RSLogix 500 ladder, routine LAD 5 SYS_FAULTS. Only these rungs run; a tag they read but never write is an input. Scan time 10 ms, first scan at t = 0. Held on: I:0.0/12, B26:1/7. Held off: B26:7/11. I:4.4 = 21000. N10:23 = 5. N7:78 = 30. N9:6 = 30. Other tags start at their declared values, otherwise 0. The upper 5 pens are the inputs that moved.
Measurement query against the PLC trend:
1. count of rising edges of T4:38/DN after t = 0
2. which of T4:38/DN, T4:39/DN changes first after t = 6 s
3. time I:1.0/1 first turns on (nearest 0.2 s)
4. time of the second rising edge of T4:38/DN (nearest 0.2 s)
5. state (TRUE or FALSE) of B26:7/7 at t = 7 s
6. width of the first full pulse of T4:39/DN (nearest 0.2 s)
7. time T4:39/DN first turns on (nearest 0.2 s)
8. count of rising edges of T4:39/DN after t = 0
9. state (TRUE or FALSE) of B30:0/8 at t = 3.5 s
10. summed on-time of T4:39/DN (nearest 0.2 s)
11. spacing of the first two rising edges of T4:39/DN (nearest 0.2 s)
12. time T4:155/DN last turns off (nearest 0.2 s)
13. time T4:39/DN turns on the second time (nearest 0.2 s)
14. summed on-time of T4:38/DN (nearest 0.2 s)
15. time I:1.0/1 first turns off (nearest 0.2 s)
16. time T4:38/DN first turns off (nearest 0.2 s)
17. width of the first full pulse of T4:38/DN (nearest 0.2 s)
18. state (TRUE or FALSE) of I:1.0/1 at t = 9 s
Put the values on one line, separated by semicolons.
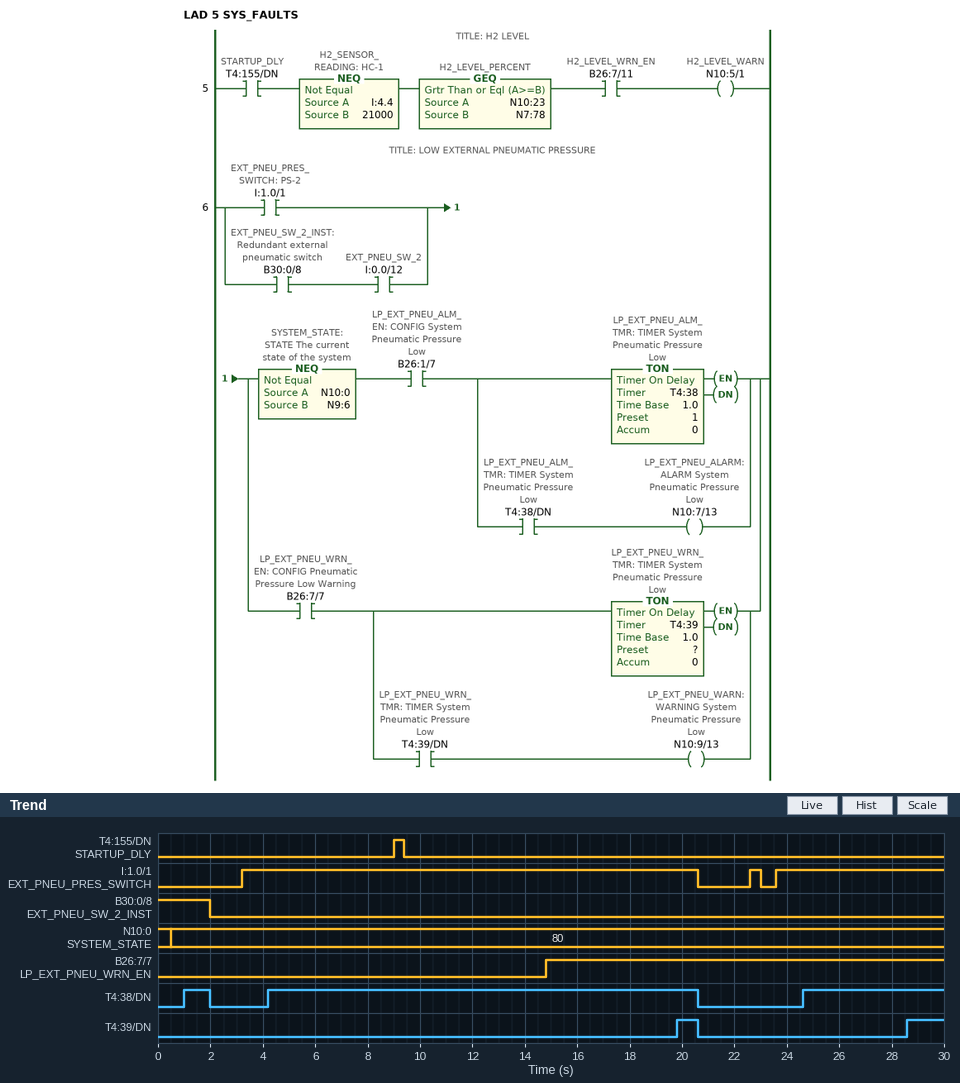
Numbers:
3; T4:39/DN; 3.2 s; 4.2 s; FALSE; 0.8 s; 19.8 s; 2; FALSE; 2.2 s; 8.8 s; 9.4 s; 28.6 s; 22.8 s; 20.6 s; 2.0 s; 1.0 s; TRUE
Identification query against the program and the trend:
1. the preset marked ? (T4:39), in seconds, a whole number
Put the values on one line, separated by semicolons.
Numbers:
5 s
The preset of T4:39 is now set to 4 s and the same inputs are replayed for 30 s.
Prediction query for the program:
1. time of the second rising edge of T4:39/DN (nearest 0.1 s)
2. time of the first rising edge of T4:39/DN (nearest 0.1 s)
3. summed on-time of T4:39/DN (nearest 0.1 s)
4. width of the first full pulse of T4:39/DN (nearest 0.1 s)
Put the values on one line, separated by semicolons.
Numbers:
27.6 s; 18.8 s; 4.2 s; 1.8 s
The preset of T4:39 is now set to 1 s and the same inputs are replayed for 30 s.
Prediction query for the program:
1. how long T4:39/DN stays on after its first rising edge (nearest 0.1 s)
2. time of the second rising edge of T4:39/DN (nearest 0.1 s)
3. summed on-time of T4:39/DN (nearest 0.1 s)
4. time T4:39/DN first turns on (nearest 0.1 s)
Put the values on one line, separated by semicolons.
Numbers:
4.8 s; 24.6 s; 10.2 s; 15.8 s
